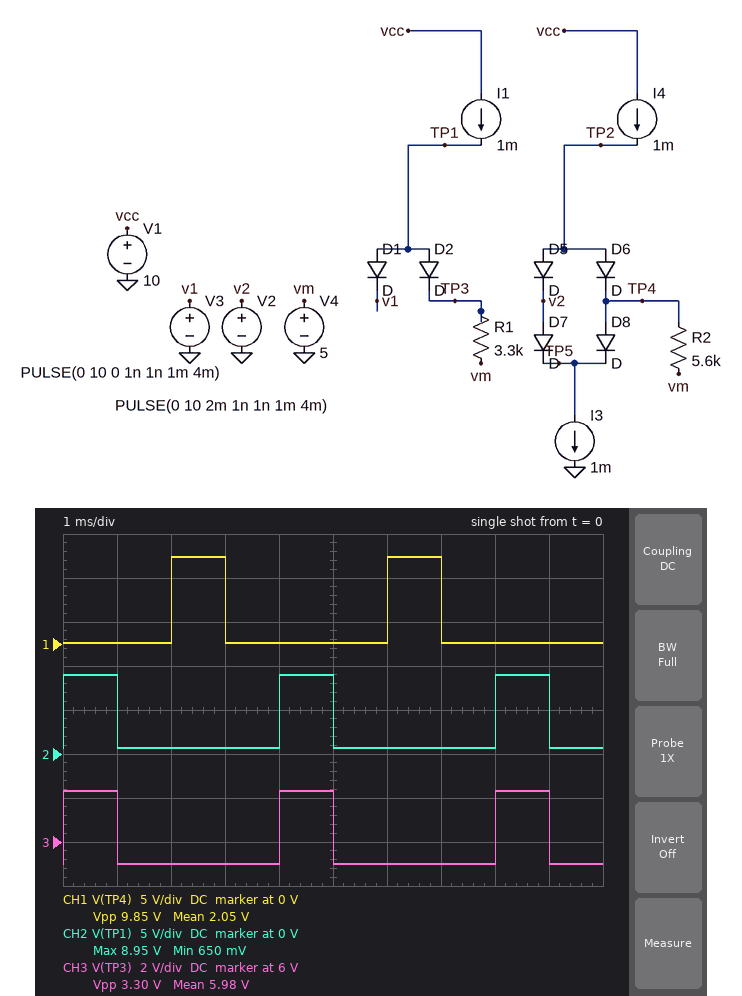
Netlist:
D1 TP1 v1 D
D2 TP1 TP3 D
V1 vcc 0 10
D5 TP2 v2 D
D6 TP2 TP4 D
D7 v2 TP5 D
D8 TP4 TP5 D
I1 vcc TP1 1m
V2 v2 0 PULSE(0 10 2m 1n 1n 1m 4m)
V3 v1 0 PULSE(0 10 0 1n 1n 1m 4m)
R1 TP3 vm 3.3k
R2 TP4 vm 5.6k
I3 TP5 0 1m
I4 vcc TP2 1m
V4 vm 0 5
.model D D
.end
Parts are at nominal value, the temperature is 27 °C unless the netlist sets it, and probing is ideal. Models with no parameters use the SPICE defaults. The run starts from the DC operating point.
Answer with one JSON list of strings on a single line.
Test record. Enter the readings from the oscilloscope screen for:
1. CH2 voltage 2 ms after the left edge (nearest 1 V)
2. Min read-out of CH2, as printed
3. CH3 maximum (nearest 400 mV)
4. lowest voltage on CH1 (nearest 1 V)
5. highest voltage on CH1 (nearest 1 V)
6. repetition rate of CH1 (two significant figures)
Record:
["1 V", "650 mV", "8.4 V", "0 V", "10 V", "250 Hz"]
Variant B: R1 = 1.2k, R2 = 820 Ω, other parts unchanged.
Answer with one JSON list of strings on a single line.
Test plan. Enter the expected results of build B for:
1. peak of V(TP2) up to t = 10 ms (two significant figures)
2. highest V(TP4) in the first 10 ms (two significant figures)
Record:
["6.5 V", "5.8 V"]
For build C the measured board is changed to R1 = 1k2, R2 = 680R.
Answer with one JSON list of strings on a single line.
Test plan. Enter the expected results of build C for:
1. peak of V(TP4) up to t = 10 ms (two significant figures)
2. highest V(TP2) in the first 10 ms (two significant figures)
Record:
["5.7 V", "6.3 V"]
